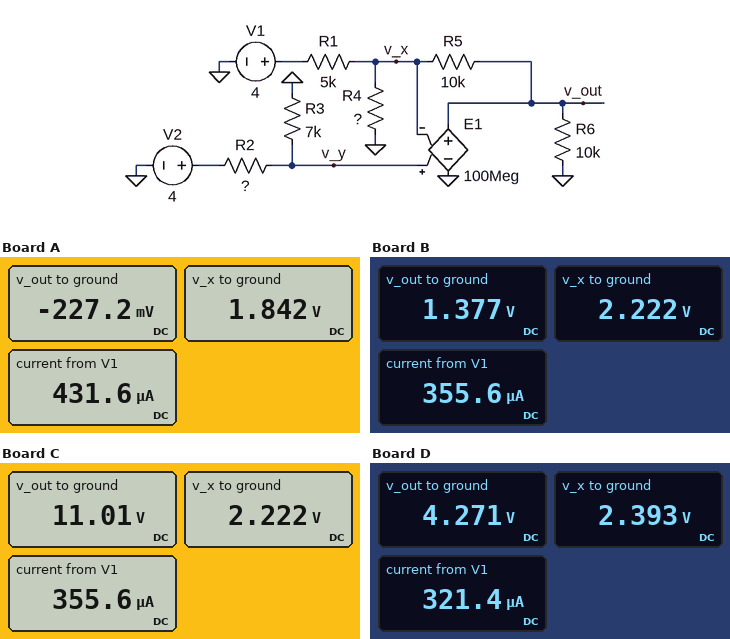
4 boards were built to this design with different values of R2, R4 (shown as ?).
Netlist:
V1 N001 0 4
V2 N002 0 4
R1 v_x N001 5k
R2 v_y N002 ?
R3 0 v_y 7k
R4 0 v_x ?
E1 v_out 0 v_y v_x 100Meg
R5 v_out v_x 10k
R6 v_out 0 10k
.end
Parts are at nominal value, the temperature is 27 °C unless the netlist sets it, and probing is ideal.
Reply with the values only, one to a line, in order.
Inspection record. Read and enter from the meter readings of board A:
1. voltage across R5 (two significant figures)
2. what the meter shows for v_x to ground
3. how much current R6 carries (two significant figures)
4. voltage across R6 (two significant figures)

2.1 V
1.842 V
23 µA
230 mV
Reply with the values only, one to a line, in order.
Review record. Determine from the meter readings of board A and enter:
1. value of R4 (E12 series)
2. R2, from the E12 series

8.2 kΩ
8.2 kΩ
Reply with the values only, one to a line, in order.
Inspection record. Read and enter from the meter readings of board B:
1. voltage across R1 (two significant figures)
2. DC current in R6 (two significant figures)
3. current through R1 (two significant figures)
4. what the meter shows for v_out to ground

1.8 V
140 µA
360 µA
1.377 V
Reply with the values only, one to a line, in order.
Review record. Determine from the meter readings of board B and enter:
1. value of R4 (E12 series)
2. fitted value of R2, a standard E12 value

8.2 kΩ
5.6 kΩ
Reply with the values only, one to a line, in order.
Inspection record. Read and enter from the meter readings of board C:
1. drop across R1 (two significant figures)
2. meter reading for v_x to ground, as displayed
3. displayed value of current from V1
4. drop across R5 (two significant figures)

1.8 V
2.222 V
355.6 µA
8.8 V
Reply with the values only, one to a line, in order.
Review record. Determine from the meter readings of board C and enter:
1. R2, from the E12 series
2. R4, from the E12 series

5.6 kΩ
1.8 kΩ
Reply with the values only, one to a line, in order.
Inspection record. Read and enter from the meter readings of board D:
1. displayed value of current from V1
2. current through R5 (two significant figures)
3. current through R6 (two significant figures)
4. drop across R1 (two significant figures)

321.4 µA
190 µA
430 µA
1.6 V
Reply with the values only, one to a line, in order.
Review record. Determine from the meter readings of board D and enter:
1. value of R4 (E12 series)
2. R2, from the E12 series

4.7 kΩ
4.7 kΩ
